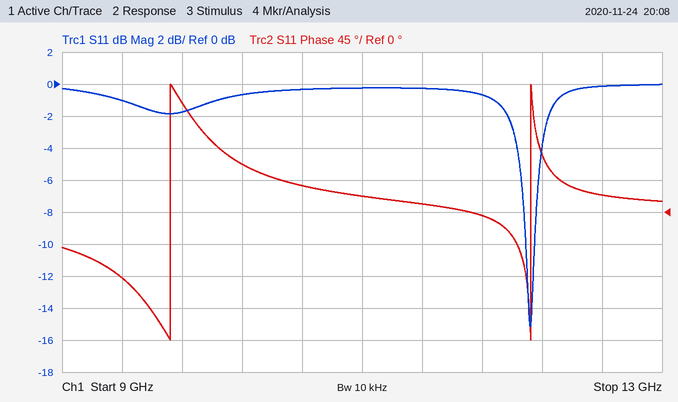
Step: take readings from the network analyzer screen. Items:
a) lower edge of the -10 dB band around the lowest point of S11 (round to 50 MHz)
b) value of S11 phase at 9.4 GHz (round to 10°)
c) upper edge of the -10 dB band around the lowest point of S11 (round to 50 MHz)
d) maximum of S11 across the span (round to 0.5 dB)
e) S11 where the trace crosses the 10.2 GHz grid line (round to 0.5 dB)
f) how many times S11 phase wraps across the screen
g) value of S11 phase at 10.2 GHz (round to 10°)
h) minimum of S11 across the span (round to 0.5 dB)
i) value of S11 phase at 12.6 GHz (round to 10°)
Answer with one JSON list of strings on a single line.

["12.10 GHz", "-90°", "12.15 GHz", "0.0 dB", "-0.5 dB", "2", "70°", "-15.0 dB", "20°"]
